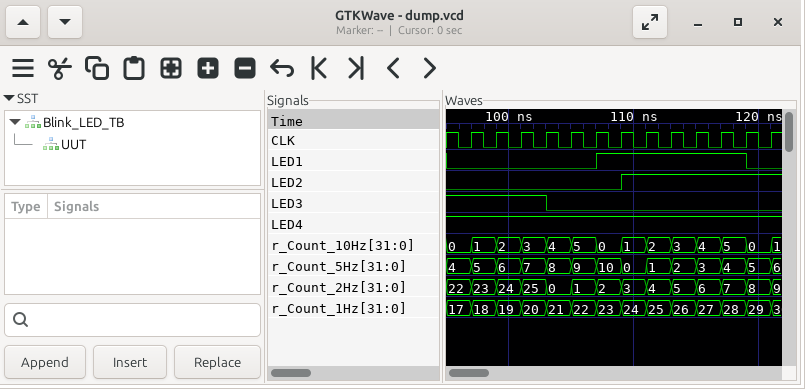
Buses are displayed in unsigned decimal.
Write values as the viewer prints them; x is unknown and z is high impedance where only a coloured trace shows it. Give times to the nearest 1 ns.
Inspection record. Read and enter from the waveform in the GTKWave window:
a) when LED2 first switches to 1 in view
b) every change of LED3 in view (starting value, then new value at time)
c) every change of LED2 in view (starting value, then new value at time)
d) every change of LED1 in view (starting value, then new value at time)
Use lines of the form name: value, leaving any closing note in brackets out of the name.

when LED2 first switches to 1 in view: 109 ns
every change of LED3 in view: 1, 0 at 103 ns
every change of LED2 in view: 0, 1 at 109 ns
every change of LED1 in view: 0, 1 at 107 ns, 0 at 119 ns
